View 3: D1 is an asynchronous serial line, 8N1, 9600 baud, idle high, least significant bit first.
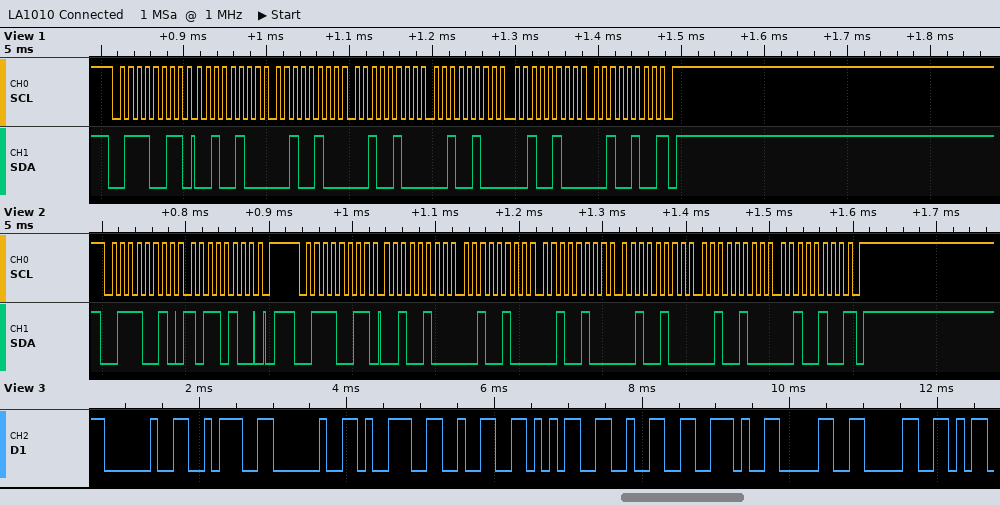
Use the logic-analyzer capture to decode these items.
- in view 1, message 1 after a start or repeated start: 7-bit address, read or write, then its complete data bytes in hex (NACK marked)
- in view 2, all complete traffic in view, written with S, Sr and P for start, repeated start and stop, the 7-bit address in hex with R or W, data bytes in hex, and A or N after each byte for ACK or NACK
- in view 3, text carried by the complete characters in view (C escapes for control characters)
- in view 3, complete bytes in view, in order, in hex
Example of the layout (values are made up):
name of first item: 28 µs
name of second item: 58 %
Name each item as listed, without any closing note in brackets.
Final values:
in view 1, message 1 after a start or repeated start: 7-bit address, read or write, then its complete data bytes in hex: 0x39 read: 24 24 24 24 24 24 NACK
in view 2, all complete traffic in view, written with S, Sr and P for start, repeated start and stop, the 7-bit address in hex with R or W, data bytes in hex, and A or N after each byte for ACK or NACK: S 39W A B4 A P S 39R A 24 A 24 A 24 A 24 A 24 A 24 N P
in view 3, text carried by the complete characters in view: " : 9252.00"
in view 3, complete bytes in view, in order, in hex: 20 3A 20 39 32 35 32 2E 30 30
